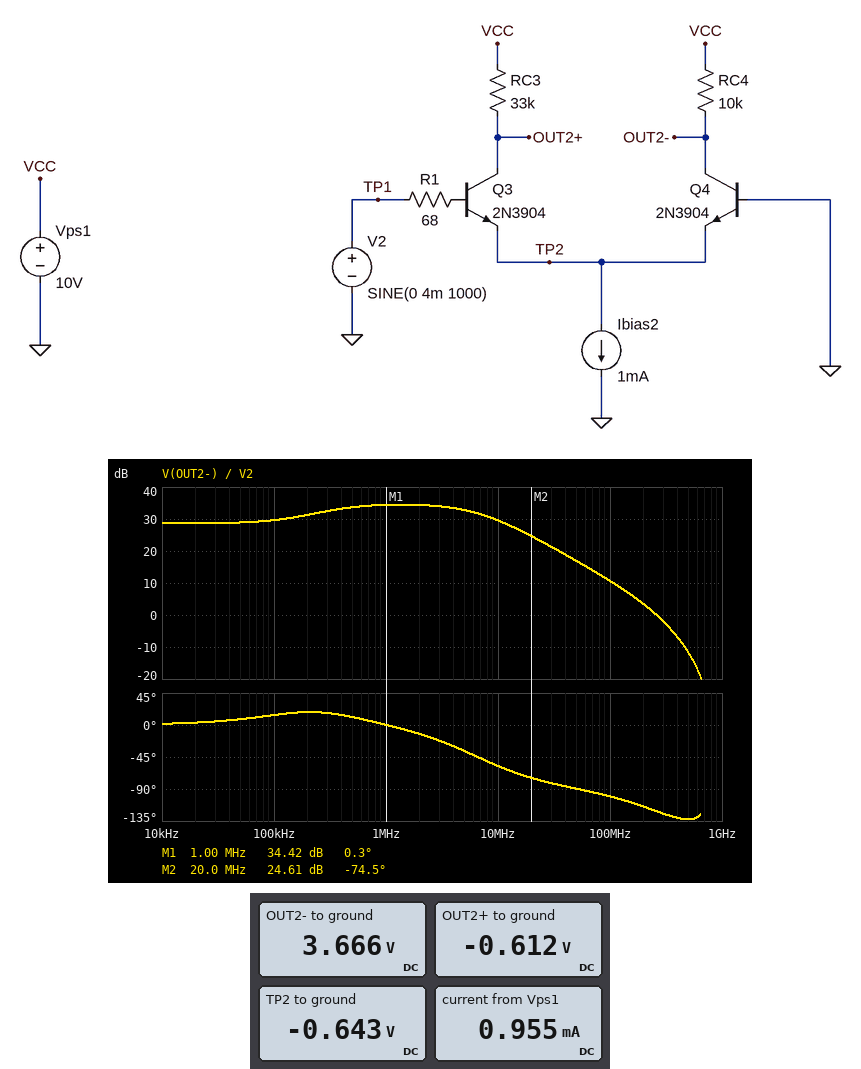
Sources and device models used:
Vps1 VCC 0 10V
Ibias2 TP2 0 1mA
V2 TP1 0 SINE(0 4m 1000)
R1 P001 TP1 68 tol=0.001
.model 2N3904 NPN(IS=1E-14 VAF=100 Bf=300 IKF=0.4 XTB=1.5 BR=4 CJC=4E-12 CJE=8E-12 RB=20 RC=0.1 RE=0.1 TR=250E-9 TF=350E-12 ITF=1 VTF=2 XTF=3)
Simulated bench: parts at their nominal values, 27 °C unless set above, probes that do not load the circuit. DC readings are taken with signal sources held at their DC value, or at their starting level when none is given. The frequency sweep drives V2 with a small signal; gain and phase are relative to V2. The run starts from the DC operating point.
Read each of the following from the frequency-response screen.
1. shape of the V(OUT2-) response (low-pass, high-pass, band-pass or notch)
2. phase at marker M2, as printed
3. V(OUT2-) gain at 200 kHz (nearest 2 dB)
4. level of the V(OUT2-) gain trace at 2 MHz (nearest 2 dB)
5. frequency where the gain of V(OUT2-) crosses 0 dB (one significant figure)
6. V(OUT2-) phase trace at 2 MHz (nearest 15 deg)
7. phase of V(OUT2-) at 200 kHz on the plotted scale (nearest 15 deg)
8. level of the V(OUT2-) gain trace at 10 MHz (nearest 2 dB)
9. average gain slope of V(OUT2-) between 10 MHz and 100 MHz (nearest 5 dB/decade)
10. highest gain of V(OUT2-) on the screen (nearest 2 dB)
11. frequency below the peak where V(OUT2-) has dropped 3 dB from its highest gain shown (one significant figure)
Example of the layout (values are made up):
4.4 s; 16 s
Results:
low-pass; -74.5 deg; 32 dB; 34 dB; 300 MHz; -15 deg; 15 deg; 30 dB; -20 dB/decade; 34 dB; 200 kHz
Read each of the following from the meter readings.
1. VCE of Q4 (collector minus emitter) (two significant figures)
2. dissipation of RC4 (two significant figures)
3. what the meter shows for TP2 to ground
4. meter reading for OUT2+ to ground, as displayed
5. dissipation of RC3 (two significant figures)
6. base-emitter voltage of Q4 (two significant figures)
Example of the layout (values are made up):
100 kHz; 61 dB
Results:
4.3 V; 4.0 mW; -0.643 V; -0.612 V; 3.4 mW; 640 mV
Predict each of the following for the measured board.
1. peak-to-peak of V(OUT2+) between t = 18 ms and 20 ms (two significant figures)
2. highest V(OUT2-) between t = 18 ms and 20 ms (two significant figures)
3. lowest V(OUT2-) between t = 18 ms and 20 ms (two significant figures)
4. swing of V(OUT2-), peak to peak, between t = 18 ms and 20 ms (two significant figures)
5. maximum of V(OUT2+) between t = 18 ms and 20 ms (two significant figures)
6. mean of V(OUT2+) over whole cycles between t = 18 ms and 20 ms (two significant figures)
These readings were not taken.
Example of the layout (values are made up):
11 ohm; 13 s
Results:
7.3 mV; 3.8 V; 3.6 V; 220 mV; -610 mV; -610 mV
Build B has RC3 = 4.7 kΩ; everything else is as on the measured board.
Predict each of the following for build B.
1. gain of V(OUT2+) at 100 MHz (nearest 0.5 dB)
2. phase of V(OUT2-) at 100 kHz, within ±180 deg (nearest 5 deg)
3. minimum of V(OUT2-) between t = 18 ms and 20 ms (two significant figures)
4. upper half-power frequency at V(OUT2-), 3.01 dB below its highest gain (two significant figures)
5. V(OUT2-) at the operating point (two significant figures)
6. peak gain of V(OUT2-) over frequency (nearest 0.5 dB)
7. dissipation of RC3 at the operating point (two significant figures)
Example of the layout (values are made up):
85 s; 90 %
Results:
12.0 dB; 0 deg; 4.7 V; 5.4 MHz; 5.1 V; 39.5 dB; 1.2 mW
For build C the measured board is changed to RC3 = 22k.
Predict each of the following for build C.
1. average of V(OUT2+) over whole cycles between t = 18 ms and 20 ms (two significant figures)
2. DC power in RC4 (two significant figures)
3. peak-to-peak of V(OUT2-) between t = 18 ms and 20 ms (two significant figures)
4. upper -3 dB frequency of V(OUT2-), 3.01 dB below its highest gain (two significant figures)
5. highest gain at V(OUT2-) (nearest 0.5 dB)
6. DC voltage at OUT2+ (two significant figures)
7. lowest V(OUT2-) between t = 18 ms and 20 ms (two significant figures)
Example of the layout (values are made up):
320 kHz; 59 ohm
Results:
-350 mV; 2.7 mW; 430 mV; 7.5 MHz; 34.0 dB; -520 mV; 4.5 V
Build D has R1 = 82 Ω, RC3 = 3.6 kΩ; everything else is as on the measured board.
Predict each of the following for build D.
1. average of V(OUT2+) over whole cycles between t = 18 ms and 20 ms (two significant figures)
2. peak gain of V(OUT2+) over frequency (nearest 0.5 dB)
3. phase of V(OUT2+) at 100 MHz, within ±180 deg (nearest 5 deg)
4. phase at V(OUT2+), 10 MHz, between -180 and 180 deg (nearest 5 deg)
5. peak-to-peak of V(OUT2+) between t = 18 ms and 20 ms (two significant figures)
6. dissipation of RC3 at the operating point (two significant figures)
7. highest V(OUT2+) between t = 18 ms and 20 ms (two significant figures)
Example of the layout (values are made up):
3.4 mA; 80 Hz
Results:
8.2 V; 30.5 dB; 70 deg; 135 deg; 270 mV; 920 µW; 8.3 V
